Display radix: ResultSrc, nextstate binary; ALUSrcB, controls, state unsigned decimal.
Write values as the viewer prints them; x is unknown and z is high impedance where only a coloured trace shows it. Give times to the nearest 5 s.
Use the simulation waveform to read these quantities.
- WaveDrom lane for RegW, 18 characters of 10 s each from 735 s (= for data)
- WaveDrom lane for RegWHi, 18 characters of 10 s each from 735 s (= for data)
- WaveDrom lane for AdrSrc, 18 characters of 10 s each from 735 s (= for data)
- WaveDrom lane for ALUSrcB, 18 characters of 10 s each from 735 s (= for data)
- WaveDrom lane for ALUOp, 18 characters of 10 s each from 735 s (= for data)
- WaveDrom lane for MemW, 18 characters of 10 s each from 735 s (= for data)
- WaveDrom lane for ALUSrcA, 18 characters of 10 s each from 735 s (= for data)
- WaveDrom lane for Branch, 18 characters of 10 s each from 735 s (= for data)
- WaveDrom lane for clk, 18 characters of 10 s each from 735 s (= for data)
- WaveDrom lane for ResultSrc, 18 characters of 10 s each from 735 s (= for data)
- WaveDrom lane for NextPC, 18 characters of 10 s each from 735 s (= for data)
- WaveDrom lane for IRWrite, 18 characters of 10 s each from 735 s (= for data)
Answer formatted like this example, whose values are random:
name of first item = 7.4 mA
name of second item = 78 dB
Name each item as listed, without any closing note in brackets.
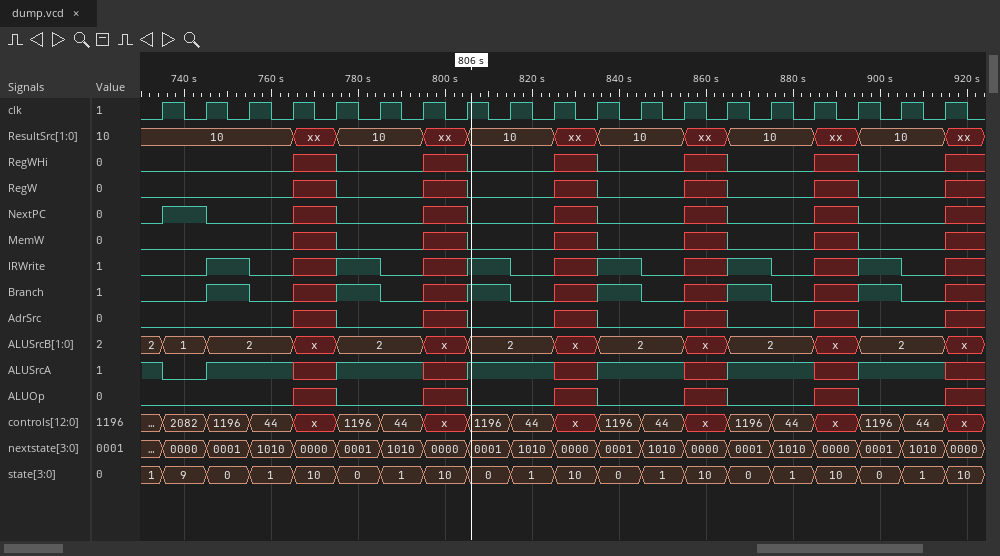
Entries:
WaveDrom lane for RegW, 18 characters of 10 s each from 735 s = {name: 'RegW', wave: '0..x0.x0.x0.x0.x0.'}
WaveDrom lane for RegWHi, 18 characters of 10 s each from 735 s = {name: 'RegWHi', wave: '0..x0.x0.x0.x0.x0.'}
WaveDrom lane for AdrSrc, 18 characters of 10 s each from 735 s = {name: 'AdrSrc', wave: '0..x0.x0.x0.x0.x0.'}
WaveDrom lane for ALUSrcB, 18 characters of 10 s each from 735 s = {name: 'ALUSrcB', wave: '==.x=.x=.x=.x=.x=.', data: '1 2 2 2 2 2 2'}
WaveDrom lane for ALUOp, 18 characters of 10 s each from 735 s = {name: 'ALUOp', wave: '0..x0.x0.x0.x0.x0.'}
WaveDrom lane for MemW, 18 characters of 10 s each from 735 s = {name: 'MemW', wave: '0..x0.x0.x0.x0.x0.'}
WaveDrom lane for ALUSrcA, 18 characters of 10 s each from 735 s = {name: 'ALUSrcA', wave: '01.x1.x1.x1.x1.x1.'}
WaveDrom lane for Branch, 18 characters of 10 s each from 735 s = {name: 'Branch', wave: '010x10x10x10x10x10'}
WaveDrom lane for clk, 18 characters of 10 s each from 735 s = {name: 'clk', wave: 'p.................'}
WaveDrom lane for ResultSrc, 18 characters of 10 s each from 735 s = {name: 'ResultSrc', wave: '=..x=.x=.x=.x=.x=.', data: '10 10 10 10 10 10'}
WaveDrom lane for NextPC, 18 characters of 10 s each from 735 s = {name: 'NextPC', wave: '10.x0.x0.x0.x0.x0.'}
WaveDrom lane for IRWrite, 18 characters of 10 s each from 735 s = {name: 'IRWrite', wave: '010x10x10x10x10x10'}
